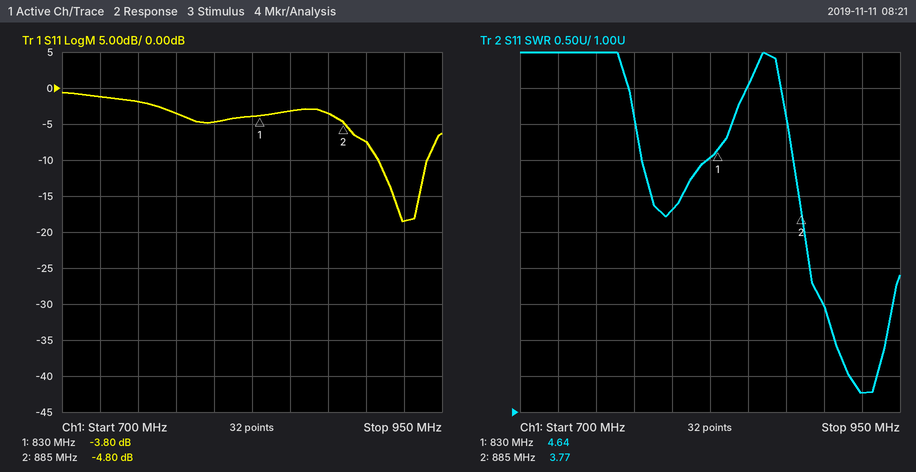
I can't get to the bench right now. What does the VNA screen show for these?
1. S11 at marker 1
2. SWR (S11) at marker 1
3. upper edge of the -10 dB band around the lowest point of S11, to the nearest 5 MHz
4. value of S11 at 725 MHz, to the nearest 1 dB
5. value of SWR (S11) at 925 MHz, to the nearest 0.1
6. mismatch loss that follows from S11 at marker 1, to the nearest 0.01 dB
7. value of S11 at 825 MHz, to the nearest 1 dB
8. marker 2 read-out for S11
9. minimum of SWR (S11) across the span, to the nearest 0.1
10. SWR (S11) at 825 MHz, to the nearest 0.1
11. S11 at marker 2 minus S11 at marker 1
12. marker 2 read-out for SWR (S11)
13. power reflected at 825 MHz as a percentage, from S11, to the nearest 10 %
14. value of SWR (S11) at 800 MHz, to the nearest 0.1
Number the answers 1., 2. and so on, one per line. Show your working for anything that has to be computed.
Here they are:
1. -3.80 dB
2. 4.64
3. 940 MHz
4. -1 dB
5. 1.3
6. −10 log10(1 − 10^(-3.8/10)) ≈ 2.34 dB
7. -4 dB
8. -4.80 dB
9. 1.3
10. 4.5
11. -4.8 − (-3.8) = -1.00 dB
12. 3.77
13. 10^(-4/10) ≈ 40 %
14. 3.8
